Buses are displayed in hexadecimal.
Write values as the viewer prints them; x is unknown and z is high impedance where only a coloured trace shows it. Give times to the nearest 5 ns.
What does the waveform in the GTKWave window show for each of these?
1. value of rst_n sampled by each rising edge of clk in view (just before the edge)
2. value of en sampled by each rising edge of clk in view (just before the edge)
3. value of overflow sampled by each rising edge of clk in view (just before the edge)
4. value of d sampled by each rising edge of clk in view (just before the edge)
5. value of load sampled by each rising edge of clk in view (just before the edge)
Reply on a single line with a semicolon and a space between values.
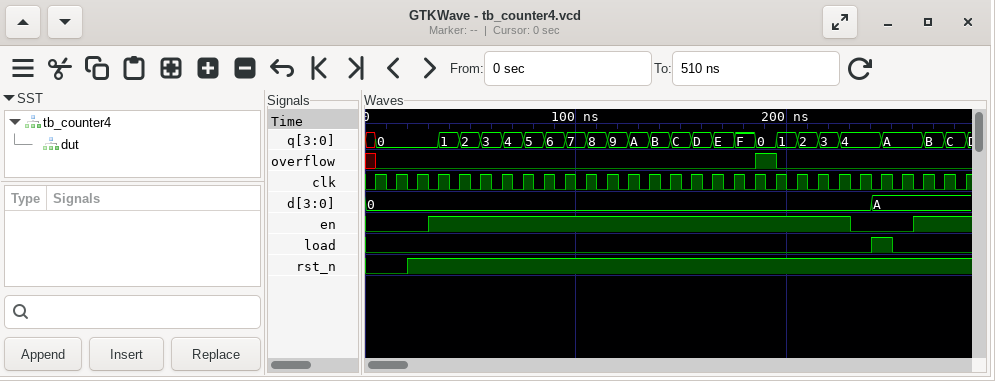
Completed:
0 0 1 1 1 1 1 1 1 1 1 1 1 1 1 1 1 1 1 1 1 1 1 1 1 1 1 1 1; 0 0 0 1 1 1 1 1 1 1 1 1 1 1 1 1 1 1 1 1 1 1 1 0 0 0 1 1 1; x 0 0 0 0 0 0 0 0 0 0 0 0 0 0 0 0 0 0 1 0 0 0 0 0 0 0 0 0; 0, 0, 0, 0, 0, 0, 0, 0, 0, 0, 0, 0, 0, 0, 0, 0, 0, 0, 0, 0, 0, 0, 0, 0, A, A, A, A, A; 0 0 0 0 0 0 0 0 0 0 0 0 0 0 0 0 0 0 0 0 0 0 0 0 1 0 0 0 0
